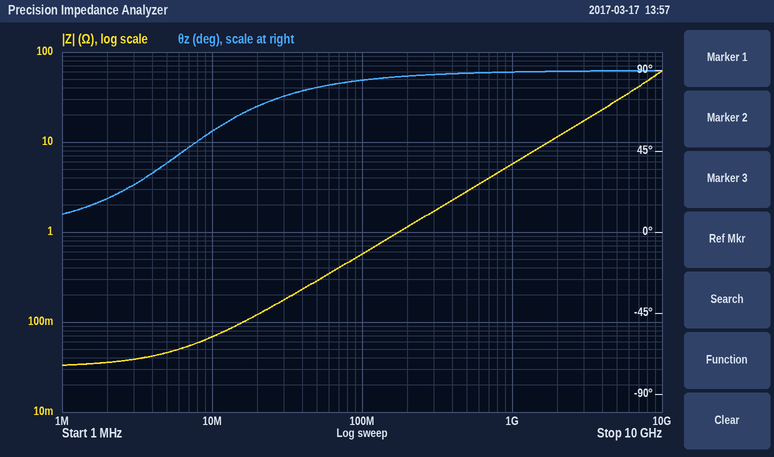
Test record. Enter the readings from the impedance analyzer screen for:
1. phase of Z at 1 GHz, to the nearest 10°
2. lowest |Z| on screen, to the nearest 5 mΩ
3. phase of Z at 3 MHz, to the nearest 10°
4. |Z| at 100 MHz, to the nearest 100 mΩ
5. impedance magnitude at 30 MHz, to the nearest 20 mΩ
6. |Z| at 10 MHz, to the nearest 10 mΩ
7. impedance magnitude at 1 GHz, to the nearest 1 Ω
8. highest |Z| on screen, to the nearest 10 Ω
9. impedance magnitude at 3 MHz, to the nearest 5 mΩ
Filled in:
90°
35 mΩ
30°
600 mΩ
180 mΩ
70 mΩ
6 Ω
60 Ω
40 mΩ
